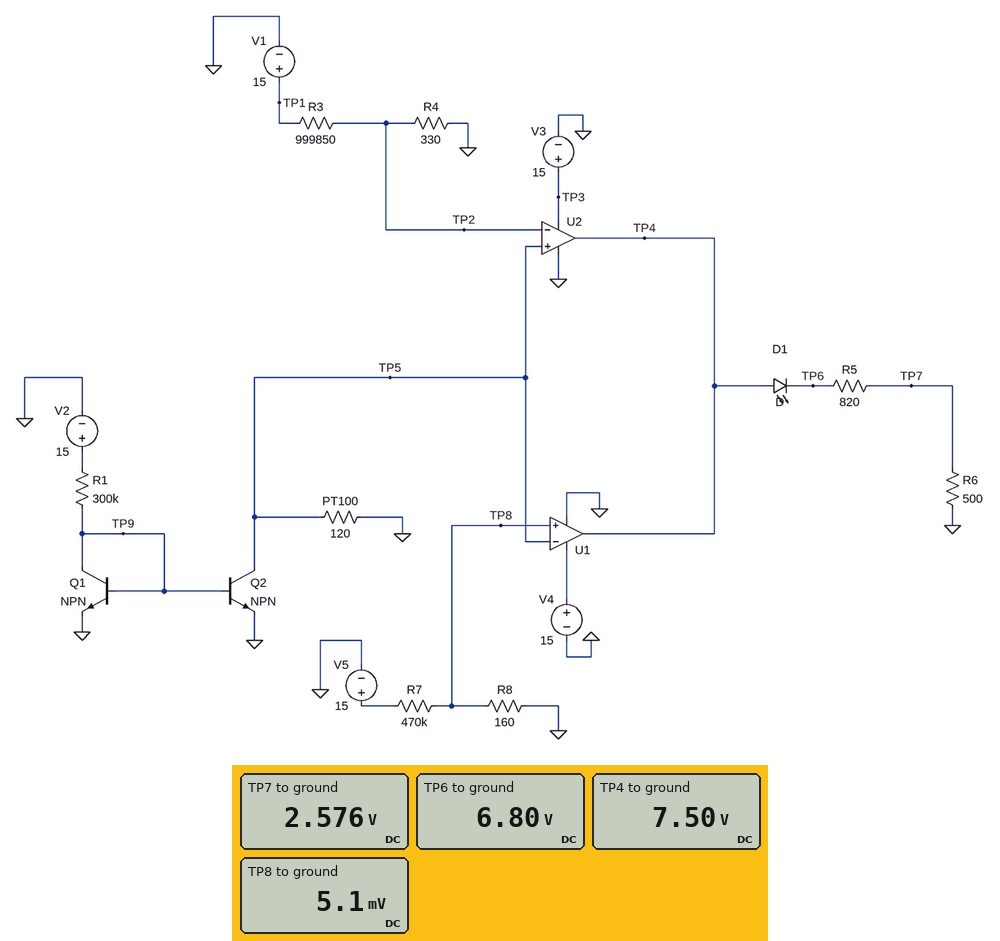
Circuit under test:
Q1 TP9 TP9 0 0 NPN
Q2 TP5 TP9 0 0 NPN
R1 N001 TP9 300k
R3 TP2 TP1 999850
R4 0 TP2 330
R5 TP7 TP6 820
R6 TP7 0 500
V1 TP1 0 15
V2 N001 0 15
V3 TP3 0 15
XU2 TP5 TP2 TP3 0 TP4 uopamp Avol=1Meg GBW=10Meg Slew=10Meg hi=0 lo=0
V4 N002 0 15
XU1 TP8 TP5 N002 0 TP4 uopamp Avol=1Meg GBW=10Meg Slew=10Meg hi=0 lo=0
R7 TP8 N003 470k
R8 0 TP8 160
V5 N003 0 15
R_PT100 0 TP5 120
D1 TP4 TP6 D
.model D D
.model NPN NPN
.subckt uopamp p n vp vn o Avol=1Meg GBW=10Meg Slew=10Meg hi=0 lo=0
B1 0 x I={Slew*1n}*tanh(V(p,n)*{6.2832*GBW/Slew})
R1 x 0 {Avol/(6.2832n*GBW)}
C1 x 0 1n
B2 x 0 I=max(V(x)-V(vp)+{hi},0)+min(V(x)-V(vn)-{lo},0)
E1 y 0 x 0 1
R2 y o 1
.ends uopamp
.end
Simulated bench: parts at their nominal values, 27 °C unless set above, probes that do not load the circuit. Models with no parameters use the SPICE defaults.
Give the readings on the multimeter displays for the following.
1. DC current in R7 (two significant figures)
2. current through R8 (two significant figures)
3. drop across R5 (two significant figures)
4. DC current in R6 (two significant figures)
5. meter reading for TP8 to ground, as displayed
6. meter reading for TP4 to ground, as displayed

32 µA
32 µA
4.2 V
5.2 mA
5.1 mV
7.50 V
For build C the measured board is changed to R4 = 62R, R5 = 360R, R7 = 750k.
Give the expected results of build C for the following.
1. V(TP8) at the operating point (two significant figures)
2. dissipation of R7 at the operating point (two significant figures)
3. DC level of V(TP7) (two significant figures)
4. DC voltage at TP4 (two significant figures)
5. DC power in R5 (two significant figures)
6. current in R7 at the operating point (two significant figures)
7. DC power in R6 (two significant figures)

3.2 mV
300 µW
8.3 V
15 V
99 mW
20 µA
140 mW
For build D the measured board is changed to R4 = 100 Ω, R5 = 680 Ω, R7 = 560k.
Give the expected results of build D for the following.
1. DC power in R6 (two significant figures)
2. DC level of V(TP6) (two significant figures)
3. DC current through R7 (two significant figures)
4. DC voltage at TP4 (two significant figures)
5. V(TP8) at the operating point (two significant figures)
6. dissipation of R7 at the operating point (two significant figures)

73 mW
14 V
27 µA
15 V
4.3 mV
400 µW
